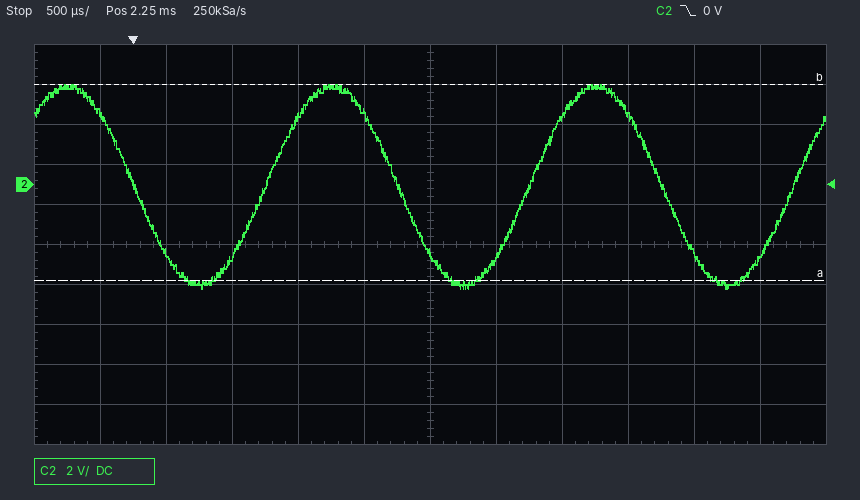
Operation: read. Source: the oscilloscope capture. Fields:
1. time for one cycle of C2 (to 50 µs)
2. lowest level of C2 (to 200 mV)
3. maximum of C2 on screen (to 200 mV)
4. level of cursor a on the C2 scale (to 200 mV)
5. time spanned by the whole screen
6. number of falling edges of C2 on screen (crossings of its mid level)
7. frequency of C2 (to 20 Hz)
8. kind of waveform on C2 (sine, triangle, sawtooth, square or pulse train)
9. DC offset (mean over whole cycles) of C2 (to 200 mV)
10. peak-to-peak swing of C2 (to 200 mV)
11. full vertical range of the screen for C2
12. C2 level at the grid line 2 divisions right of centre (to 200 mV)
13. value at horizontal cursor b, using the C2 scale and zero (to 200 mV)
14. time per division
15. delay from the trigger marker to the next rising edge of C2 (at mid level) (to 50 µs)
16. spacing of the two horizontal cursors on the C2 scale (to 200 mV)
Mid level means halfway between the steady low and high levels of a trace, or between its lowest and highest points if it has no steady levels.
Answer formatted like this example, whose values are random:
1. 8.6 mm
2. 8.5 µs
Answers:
1. 2.00 ms
2. -5.2 V
3. 5.0 V
4. -4.8 V
5. 6 ms
6. 3
7. 500 Hz
8. sine
9. 0.0 V
10. 10.2 V
11. 20 V
12. 3.4 V
13. 5.0 V
14. 500 µs
15. 1.00 ms
16. 9.8 V
